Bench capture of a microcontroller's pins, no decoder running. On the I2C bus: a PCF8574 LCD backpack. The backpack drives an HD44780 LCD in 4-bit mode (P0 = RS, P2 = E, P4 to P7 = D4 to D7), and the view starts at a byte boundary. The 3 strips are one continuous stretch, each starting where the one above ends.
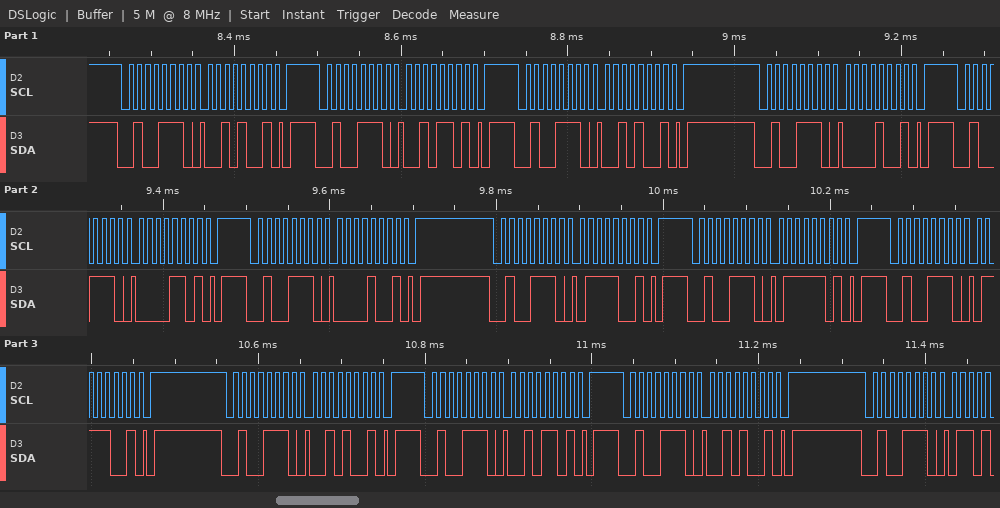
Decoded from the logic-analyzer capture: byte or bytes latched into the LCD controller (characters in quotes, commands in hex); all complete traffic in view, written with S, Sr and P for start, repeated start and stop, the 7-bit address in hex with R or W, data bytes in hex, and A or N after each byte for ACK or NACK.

' ' 'r'
S 27W A 29 A P S 27W A 2D A P S 27W A 29 A P S 27W A 09 A P S 27W A 0D A P S 27W A 09 A P S 27W A 79 A P S 27W A 7D A P S 27W A 79 A P S 27W A 29 A P S 27W A 2D A P S 27W A 29 A P S 27W A
